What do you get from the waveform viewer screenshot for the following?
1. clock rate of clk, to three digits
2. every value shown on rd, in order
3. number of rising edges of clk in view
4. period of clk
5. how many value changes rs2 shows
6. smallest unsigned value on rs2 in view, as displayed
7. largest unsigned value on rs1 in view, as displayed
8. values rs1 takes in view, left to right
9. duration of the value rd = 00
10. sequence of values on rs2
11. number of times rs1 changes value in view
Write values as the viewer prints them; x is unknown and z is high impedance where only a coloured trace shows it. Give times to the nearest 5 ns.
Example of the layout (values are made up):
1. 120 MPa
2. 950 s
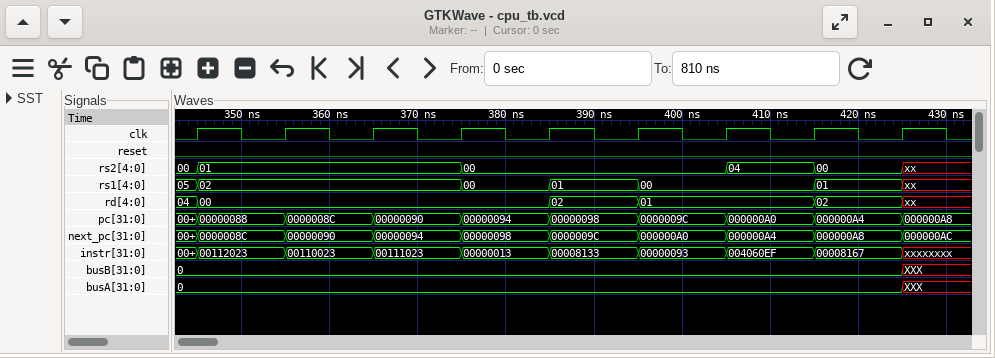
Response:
1. 100 MHz
2. 04, 00, 02, 01, 02, xx
3. 9
4. 10 ns
5. 5
6. 00
7. 05
8. 05, 02, 00, 01, 00, 01, xx
9. 40 ns
10. 00, 01, 00, 04, 00, xx
11. 6
